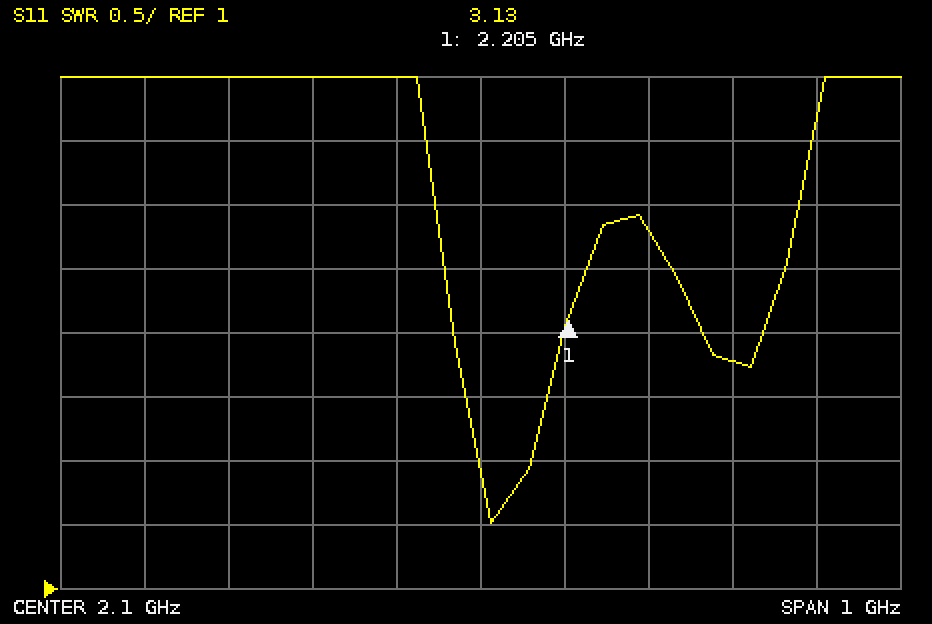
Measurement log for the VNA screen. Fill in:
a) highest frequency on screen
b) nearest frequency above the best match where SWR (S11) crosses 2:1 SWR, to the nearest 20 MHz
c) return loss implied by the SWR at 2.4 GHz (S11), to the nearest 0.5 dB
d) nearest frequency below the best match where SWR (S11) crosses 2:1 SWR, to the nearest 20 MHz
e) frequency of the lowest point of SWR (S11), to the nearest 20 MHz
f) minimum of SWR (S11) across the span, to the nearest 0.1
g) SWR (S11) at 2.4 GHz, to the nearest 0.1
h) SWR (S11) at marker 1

2.6 GHz
2.16 GHz
6.5 dB
2.10 GHz
2.12 GHz
1.5
2.8
3.13
